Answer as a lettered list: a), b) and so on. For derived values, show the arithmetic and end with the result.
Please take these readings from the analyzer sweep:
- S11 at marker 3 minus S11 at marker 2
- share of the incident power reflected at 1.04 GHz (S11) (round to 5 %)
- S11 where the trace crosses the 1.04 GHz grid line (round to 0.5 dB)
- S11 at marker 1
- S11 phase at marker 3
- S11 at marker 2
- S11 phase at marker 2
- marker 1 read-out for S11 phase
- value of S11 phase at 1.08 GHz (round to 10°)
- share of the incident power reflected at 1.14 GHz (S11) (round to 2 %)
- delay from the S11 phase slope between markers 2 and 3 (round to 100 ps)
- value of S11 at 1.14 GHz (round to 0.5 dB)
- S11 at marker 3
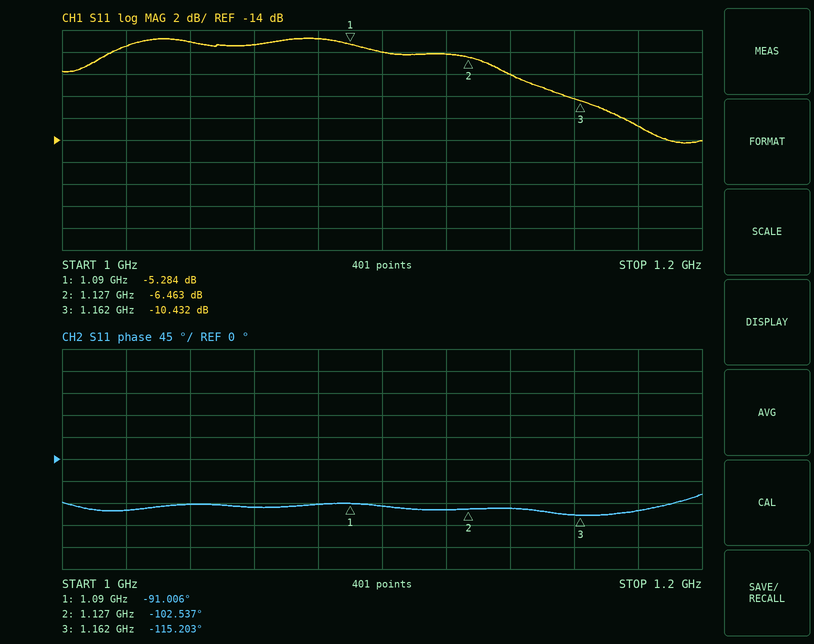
a) -10.432 − (-6.463) = -3.969 dB
b) 10^(-5/10) ≈ 31.6 %, so 30 % to the nearest 5 %
c) -5.0 dB
d) -5.284 dB
e) -115.203°
f) -6.463 dB
g) -102.537°
h) -91.006°
i) -90°
j) 10^(-8/10) ≈ 16 %
k) −(-115.203° − (-102.537°))/(360° × 35 MHz) ≈ 1.0 ns
l) -8.0 dB
m) -10.432 dB
